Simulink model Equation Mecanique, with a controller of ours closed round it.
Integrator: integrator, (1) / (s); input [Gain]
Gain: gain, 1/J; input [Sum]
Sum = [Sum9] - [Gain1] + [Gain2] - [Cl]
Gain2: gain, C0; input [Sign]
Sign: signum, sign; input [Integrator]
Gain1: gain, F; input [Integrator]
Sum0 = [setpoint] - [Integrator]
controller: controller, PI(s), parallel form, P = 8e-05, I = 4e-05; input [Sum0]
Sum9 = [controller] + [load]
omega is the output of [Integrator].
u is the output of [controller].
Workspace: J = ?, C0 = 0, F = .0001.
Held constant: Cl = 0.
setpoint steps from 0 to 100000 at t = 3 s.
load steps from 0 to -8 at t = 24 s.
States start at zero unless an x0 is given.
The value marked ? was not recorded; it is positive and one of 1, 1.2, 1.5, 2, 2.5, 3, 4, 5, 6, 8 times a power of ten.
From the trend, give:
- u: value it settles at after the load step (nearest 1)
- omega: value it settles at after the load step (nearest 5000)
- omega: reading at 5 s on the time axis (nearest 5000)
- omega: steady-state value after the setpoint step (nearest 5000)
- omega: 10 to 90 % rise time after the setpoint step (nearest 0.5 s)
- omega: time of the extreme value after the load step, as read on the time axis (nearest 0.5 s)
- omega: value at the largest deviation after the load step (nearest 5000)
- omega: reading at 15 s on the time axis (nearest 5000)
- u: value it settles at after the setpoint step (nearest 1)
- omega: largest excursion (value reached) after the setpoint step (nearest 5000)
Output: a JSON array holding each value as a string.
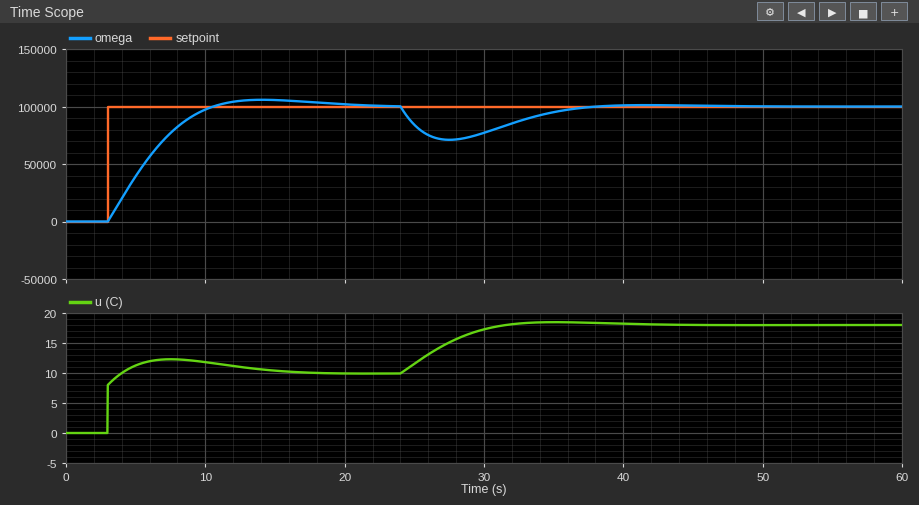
["18", "100000", "40000", "100000", "5.5 s", "27.5 s", "70000", "105000", "10", "105000"]
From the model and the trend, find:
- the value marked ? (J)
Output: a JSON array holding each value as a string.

["0.0004"]
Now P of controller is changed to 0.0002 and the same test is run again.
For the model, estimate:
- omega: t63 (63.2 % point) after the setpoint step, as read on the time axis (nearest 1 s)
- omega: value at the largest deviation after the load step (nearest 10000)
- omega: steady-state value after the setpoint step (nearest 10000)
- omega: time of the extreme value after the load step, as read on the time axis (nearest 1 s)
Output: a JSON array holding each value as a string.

["5 s", "80000", "100000", "27 s"]
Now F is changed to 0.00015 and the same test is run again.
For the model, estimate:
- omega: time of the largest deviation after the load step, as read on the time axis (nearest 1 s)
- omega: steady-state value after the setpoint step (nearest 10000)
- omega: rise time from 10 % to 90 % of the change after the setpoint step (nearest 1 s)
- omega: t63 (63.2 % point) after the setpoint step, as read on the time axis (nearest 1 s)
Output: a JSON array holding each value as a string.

["27 s", "100000", "8 s", "7 s"]
